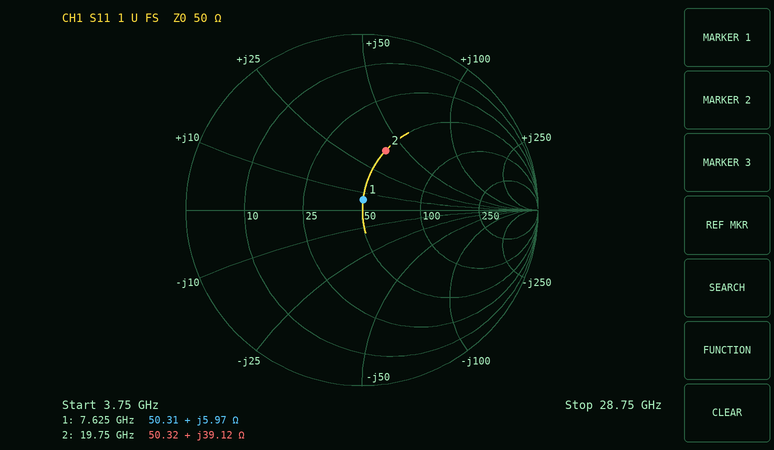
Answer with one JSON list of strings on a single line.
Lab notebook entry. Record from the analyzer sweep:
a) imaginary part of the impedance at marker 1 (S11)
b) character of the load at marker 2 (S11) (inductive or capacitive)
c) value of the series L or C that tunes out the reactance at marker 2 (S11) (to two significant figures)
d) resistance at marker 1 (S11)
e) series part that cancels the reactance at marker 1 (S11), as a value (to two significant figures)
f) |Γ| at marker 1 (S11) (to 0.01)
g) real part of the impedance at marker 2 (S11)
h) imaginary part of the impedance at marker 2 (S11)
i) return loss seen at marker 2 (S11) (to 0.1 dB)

["+5.97 Ω", "inductive", "210 fF", "50.31 Ω", "3.5 pF", "0.06", "50.32 Ω", "+39.12 Ω", "8.8 dB"]
